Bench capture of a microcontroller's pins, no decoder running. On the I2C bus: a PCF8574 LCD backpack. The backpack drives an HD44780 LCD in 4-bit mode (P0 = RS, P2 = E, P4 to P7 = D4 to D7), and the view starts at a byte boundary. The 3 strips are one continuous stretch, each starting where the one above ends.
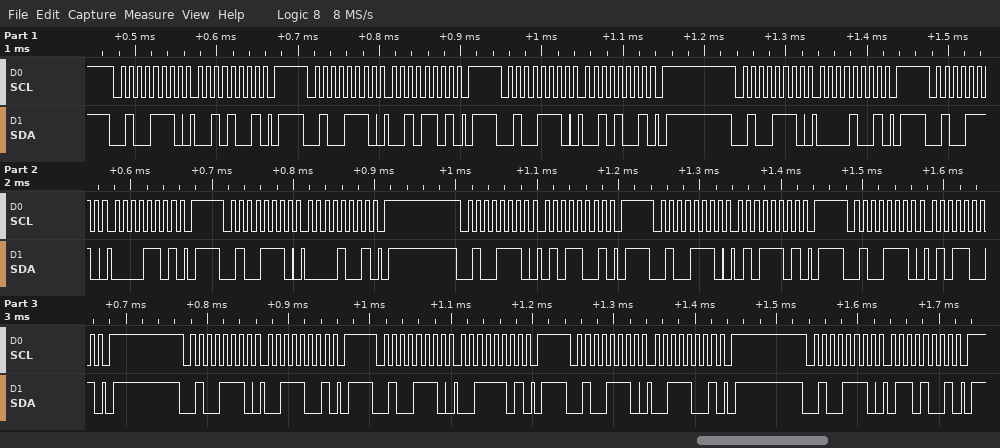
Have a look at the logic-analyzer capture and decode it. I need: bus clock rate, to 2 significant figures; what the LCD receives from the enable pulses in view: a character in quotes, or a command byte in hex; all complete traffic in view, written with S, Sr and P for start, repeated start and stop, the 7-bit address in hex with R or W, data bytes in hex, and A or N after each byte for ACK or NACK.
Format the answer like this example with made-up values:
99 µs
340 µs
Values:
100 kHz
' ' 'S'
S 27W A 29 A P S 27W A 2D A P S 27W A 29 A P S 27W A 09 A P S 27W A 0D A P S 27W A 09 A P S 27W A 59 A P S 27W A 5D A P S 27W A 59 A P S 27W A 39 A P S 27W A 3D A P S 27W A 39 A P S 27W A 69 A P
